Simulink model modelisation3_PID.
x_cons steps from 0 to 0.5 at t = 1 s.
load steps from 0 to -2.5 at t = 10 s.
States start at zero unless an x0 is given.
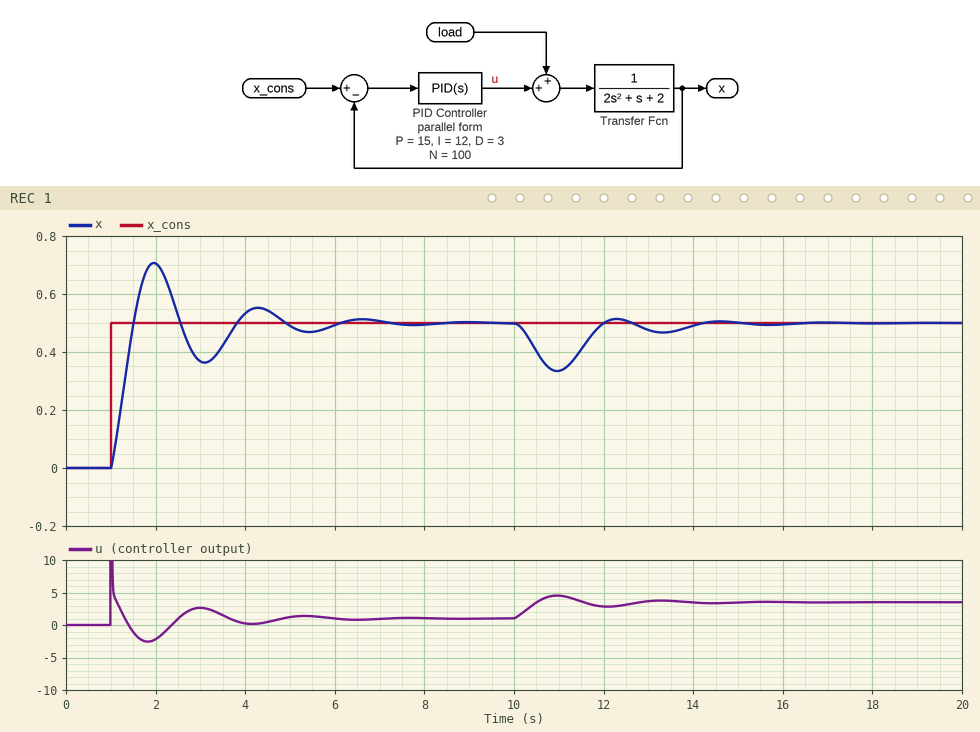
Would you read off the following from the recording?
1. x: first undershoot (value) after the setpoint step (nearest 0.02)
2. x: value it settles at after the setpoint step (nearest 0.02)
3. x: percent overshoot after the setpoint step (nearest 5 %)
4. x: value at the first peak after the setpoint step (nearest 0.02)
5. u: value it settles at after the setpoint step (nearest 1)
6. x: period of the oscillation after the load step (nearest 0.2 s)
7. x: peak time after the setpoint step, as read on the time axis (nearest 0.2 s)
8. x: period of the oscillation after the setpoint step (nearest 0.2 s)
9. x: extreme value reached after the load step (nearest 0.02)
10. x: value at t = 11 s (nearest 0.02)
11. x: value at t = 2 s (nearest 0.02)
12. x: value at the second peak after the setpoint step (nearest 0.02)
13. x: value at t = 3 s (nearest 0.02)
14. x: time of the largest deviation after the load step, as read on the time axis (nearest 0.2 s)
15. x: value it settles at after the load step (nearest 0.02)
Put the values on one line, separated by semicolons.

0.36; 0.50; 40 %; 0.70; 1; 2.4 s; 2.0 s; 2.4 s; 0.34; 0.34; 0.70; 0.56; 0.36; 11.0 s; 0.50
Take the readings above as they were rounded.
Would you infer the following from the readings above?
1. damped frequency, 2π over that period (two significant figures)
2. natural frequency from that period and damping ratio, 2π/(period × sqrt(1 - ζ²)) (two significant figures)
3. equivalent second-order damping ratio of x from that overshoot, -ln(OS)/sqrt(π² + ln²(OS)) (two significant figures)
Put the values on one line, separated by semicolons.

2.6 rad/s; 2.7 rad/s; 0.28
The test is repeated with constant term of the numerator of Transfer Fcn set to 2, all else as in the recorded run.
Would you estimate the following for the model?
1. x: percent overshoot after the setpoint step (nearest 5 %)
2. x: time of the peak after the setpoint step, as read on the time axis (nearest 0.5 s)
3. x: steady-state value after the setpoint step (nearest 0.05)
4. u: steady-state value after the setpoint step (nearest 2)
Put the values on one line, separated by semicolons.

35 %; 1.5 s; 0.50; 0
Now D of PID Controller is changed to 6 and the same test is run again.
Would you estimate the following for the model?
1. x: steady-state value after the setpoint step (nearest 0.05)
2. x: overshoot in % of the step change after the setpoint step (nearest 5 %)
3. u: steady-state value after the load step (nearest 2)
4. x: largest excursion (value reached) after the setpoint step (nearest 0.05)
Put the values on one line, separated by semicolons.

0.50; 20 %; 4; 0.60
